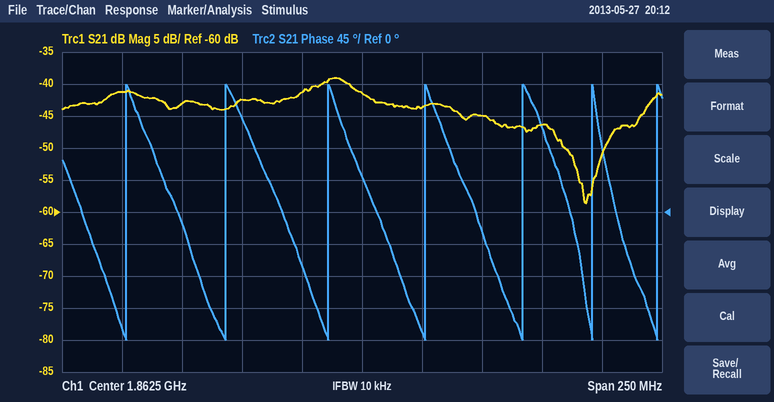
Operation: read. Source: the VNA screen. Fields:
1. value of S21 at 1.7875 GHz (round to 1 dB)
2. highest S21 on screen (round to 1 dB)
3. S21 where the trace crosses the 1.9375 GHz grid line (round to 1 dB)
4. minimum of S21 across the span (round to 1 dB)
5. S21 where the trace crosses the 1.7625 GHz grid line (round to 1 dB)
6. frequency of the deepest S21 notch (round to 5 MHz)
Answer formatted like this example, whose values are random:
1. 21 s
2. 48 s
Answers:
1. -43 dB
2. -39 dB
3. -46 dB
4. -59 dB
5. -41 dB
6. 1.955 GHz
